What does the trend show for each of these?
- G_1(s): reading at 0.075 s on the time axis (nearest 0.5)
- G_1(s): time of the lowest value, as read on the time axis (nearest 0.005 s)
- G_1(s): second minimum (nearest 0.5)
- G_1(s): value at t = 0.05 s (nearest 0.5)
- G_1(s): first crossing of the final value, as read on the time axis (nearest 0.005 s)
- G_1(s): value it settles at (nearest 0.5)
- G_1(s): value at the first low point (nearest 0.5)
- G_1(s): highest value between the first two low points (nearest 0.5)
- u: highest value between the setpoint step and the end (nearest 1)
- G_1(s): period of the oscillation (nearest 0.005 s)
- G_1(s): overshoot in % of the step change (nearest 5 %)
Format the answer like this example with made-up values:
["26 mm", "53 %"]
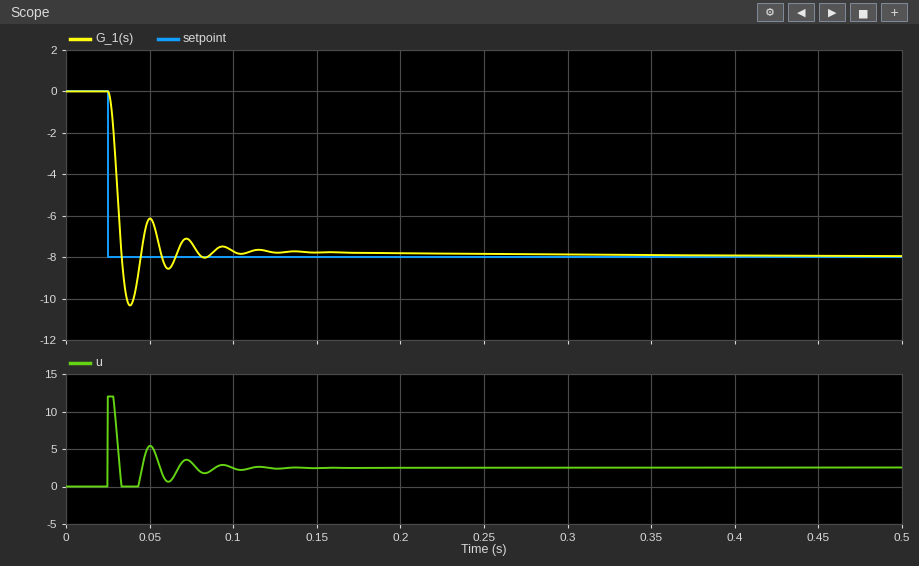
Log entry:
["-7.5", "0.040 s", "-8.5", "-6.0", "0.035 s", "-8.0", "-10.5", "-6.0", "12", "0.025 s", "30 %"]
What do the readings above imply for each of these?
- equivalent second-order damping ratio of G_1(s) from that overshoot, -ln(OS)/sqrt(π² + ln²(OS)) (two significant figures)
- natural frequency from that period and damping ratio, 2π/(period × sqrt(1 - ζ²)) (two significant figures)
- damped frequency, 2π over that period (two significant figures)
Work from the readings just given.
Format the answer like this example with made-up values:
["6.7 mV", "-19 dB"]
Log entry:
["0.36", "270 rad/s", "250 rad/s"]
